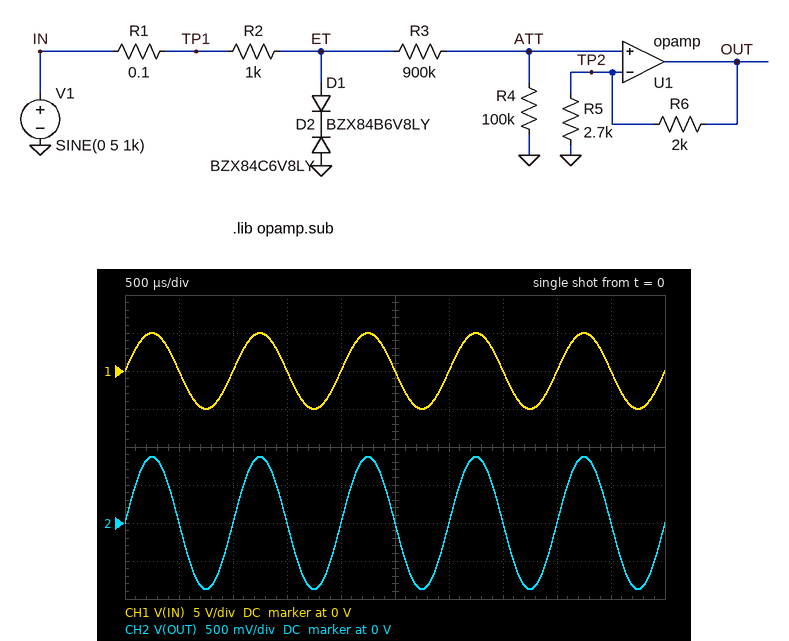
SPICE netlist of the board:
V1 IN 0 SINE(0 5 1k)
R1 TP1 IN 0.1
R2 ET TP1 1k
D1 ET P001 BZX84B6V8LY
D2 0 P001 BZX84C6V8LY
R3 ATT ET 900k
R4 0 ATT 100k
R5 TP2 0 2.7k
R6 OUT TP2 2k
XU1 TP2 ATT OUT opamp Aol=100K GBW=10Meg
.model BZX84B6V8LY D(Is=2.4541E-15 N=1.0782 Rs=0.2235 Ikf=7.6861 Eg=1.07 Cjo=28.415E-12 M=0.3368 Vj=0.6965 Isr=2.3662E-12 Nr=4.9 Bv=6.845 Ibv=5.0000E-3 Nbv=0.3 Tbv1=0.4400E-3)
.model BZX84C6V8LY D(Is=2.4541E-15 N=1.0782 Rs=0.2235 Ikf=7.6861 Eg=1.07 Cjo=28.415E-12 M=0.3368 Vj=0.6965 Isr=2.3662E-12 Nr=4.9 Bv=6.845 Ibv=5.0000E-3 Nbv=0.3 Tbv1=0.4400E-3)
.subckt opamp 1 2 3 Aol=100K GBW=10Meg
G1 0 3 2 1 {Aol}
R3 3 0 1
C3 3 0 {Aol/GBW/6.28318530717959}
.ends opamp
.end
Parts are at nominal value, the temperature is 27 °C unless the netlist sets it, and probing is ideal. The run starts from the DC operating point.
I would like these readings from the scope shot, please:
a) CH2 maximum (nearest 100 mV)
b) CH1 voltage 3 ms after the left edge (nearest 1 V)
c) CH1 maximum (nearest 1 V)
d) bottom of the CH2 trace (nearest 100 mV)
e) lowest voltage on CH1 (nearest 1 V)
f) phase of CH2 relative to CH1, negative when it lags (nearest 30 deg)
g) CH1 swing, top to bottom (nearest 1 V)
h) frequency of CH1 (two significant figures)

900 mV
0 V
5 V
-900 mV
-5 V
0 deg
10 V
1.0 kHz
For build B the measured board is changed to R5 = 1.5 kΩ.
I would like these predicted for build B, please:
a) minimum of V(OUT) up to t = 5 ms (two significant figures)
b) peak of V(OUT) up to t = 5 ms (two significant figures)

-1.2 V
1.2 V
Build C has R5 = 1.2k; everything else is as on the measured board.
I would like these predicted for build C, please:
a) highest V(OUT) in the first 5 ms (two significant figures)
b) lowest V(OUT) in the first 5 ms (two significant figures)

1.3 V
-1.3 V
